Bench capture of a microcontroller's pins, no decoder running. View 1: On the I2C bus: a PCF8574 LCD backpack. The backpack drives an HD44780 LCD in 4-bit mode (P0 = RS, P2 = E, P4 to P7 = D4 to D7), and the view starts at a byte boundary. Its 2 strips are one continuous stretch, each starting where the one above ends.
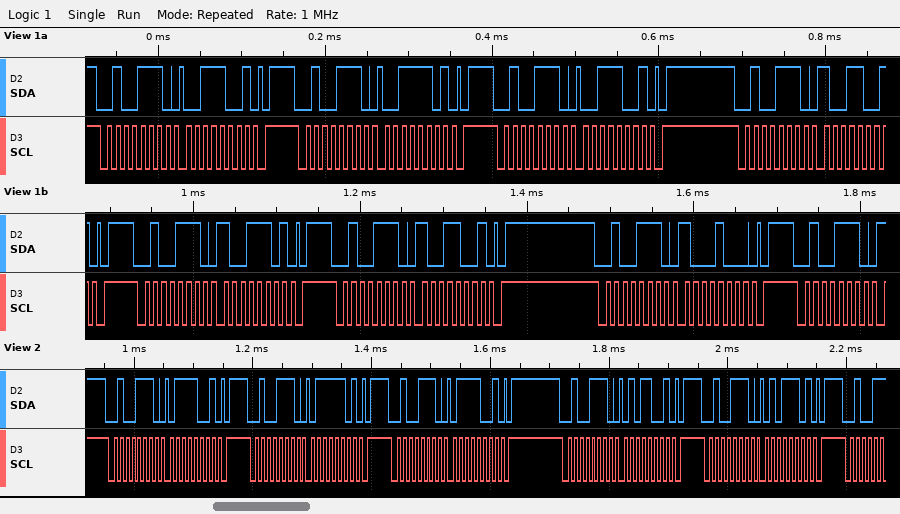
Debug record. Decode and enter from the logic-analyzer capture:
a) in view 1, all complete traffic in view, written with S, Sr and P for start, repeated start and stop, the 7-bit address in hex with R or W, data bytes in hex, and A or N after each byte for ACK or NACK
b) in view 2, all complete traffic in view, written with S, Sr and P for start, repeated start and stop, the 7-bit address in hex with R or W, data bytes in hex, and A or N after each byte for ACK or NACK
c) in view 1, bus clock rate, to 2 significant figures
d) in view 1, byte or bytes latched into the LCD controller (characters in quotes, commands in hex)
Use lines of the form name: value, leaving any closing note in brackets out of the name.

in view 1, all complete traffic in view, written with S, Sr and P for start, repeated start and stop, the 7-bit address in hex with R or W, data bytes in hex, and A or N after each byte for ACK or NACK: S 27W A 39 A P S 27W A 3D A P S 27W A 39 A P S 27W A 99 A P S 27W A 9D A P S 27W A 99 A P S 27W A 88 A P S 27W A
in view 2, all complete traffic in view, written with S, Sr and P for start, repeated start and stop, the 7-bit address in hex with R or W, data bytes in hex, and A or N after each byte for ACK or NACK: S 27W A 79 A P S 27W A 7D A P S 27W A 79 A P S 27W A 59 A P S 27W A 5D A P
in view 1, bus clock rate, to 2 significant figures: 100 kHz
in view 1, byte or bytes latched into the LCD controller: '9'
